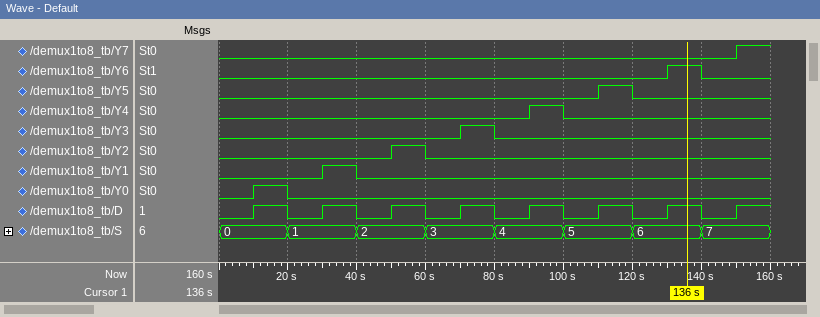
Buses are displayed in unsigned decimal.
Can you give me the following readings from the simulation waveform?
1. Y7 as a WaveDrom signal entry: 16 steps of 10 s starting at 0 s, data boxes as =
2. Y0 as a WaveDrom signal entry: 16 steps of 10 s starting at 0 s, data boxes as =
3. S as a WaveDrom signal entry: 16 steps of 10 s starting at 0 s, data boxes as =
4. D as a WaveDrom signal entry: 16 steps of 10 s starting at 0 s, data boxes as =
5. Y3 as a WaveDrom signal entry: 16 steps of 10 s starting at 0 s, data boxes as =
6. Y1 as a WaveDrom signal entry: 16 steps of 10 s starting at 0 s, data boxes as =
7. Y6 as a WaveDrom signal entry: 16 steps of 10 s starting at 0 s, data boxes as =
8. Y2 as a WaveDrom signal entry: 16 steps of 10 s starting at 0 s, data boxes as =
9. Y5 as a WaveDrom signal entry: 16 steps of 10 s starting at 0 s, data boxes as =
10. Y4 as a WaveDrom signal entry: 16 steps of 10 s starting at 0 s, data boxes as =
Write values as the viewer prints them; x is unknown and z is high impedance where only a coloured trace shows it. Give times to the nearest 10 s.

{name: 'Y7', wave: '0..............1'}
{name: 'Y0', wave: '010.............'}
{name: 'S', wave: '=.=.=.=.=.=.=.=.', data: '0 1 2 3 4 5 6 7'}
{name: 'D', wave: '0101010101010101'}
{name: 'Y3', wave: '0......10.......'}
{name: 'Y1', wave: '0..10...........'}
{name: 'Y6', wave: '0............10.'}
{name: 'Y2', wave: '0....10.........'}
{name: 'Y5', wave: '0..........10...'}
{name: 'Y4', wave: '0........10.....'}
